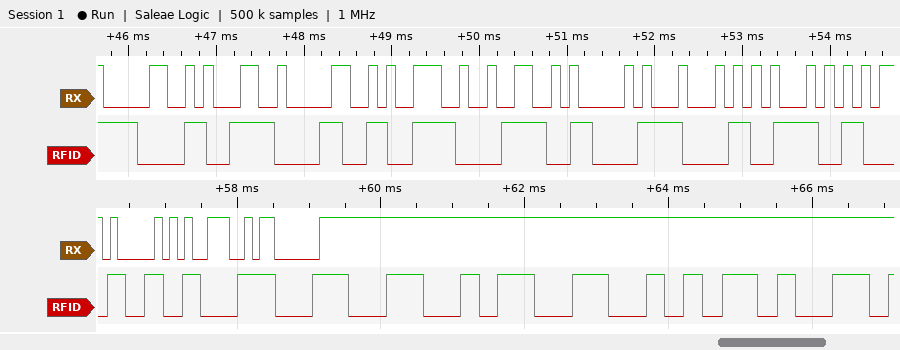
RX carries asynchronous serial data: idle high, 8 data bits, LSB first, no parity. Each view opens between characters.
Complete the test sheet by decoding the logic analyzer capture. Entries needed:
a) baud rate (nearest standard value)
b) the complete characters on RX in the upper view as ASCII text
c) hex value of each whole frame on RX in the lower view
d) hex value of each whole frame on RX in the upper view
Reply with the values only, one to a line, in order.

9600 baud
"01092ADE"
41, 39, 03
30, 31, 30, 39, 32, 41, 44, 45
